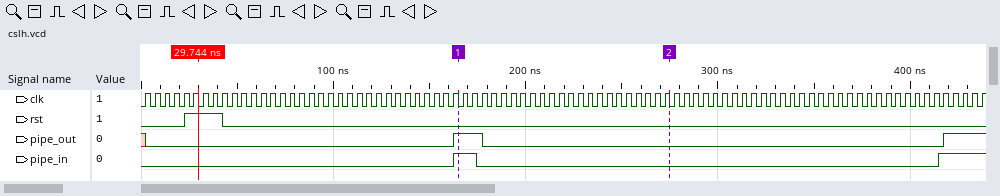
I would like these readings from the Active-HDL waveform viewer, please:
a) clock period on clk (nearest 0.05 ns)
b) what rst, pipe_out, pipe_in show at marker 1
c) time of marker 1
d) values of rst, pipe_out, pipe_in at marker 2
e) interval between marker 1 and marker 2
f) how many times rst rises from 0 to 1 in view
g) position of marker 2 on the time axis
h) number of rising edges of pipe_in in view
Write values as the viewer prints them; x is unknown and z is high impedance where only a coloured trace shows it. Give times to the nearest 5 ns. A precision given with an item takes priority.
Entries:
5 ns
rst=0, pipe_out=1, pipe_in=1
165 ns
rst=0, pipe_out=0, pipe_in=0
110 ns
1
275 ns
2
